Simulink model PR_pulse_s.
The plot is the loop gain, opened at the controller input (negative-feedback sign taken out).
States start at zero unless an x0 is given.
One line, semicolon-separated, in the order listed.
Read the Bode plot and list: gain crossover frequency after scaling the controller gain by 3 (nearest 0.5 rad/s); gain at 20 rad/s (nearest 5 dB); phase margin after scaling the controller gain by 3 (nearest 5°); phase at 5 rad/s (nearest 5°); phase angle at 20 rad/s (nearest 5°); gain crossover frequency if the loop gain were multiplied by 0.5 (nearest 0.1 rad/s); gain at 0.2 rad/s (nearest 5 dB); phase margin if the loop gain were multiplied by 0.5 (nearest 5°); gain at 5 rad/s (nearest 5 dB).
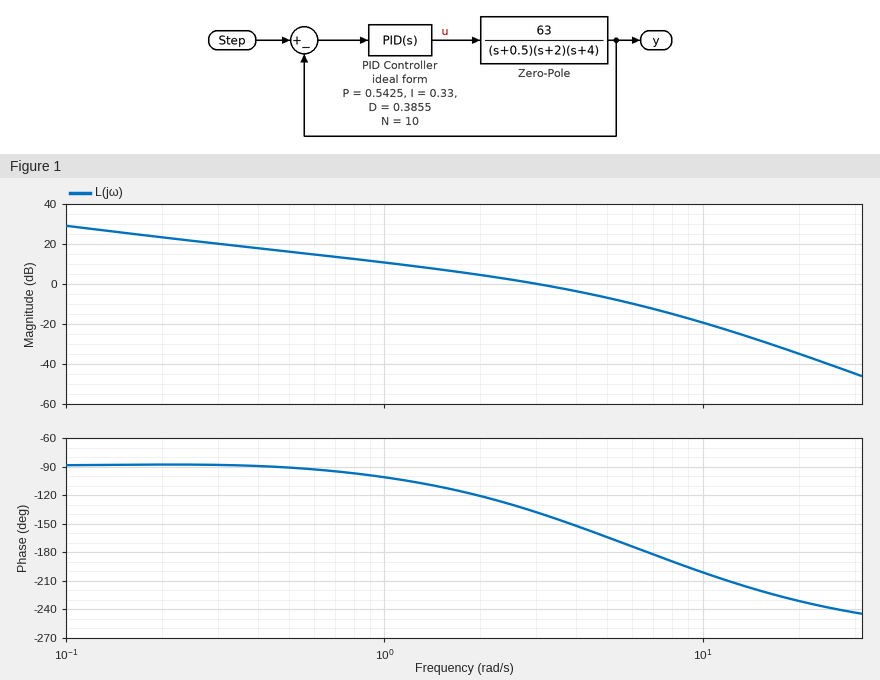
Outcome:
6.0 rad/s; -35 dB; 5°; -165°; -230°; 1.7 rad/s; 25 dB; 65°; -5 dB
